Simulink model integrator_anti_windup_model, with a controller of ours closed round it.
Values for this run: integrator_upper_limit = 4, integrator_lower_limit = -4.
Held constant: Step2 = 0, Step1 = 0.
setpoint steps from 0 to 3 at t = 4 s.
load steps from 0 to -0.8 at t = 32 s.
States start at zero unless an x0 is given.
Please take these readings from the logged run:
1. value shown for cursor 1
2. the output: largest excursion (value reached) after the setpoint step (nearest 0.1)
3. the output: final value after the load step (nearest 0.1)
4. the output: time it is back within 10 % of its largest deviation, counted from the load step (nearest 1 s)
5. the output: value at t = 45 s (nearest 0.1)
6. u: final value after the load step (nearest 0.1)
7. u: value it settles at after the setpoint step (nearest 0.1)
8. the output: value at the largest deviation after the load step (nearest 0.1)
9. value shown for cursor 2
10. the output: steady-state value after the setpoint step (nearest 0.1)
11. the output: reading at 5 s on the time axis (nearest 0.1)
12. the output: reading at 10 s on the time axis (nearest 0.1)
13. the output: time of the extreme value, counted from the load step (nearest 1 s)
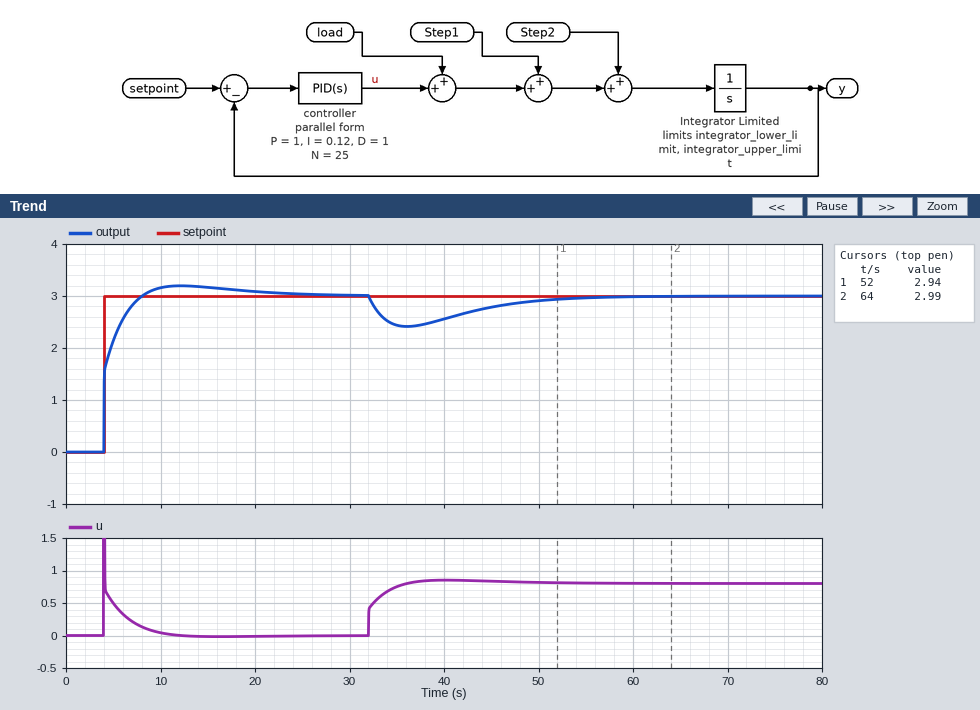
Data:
2.94
3.2
3.0
20 s
2.8
0.8
0.0
2.4
2.99
3.0
2.1
3.2
4 s
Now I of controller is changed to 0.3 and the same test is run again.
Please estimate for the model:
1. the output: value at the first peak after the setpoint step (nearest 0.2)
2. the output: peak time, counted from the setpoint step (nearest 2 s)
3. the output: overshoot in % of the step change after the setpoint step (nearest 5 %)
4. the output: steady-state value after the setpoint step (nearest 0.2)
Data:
3.4
6 s
10 %
3.0
